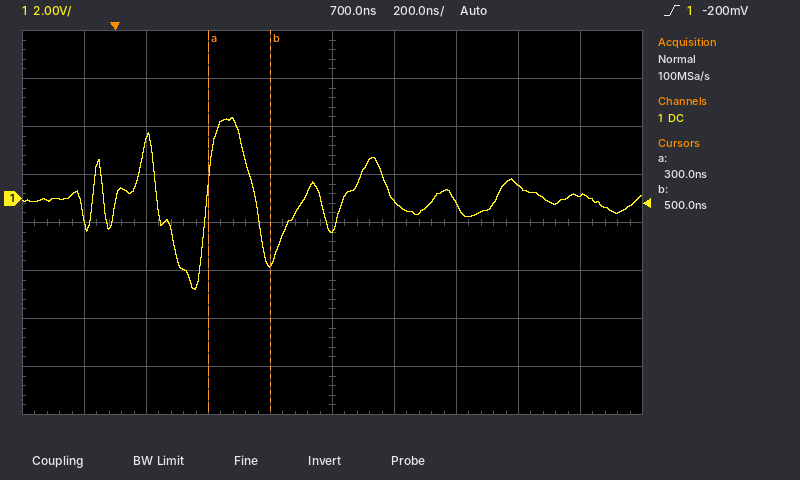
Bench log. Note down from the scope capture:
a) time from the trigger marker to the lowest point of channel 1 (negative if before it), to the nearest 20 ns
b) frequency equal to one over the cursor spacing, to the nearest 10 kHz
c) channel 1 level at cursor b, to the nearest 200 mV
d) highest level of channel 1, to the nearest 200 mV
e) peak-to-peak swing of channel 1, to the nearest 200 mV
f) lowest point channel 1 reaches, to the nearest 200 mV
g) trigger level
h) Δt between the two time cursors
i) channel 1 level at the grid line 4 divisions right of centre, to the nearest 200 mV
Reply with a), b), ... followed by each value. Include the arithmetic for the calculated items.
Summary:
a) +260 ns
b) 1 / 200 ns ≈ 5.00 MHz
c) -2.6 V
d) 3.4 V
e) 3.4 V − (-3.8 V) = 7.2 V
f) -3.8 V
g) -200 mV
h) 500 ns − (300 ns) = 200 ns
i) 200 mV
